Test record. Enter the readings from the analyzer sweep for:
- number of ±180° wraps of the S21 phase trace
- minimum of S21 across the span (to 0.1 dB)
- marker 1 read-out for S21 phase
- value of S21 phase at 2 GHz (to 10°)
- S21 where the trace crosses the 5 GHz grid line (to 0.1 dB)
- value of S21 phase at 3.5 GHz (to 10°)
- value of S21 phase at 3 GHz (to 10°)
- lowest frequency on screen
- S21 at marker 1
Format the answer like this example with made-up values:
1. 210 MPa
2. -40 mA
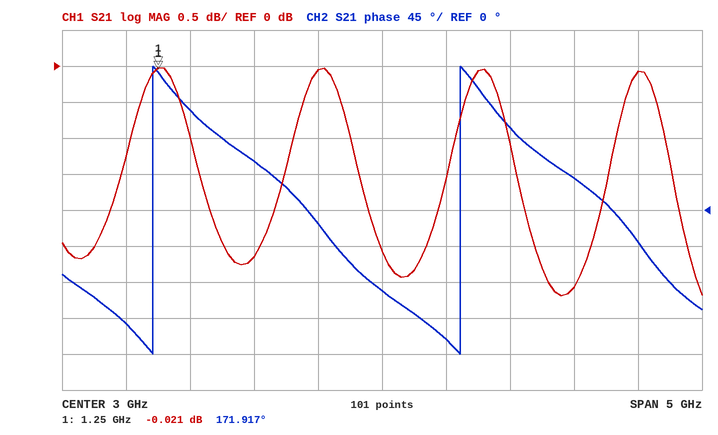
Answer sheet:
1. 2
2. -3.2 dB
3. 171.917°
4. 60°
5. -0.1 dB
6. -160°
7. -100°
8. 500 MHz
9. -0.021 dB
